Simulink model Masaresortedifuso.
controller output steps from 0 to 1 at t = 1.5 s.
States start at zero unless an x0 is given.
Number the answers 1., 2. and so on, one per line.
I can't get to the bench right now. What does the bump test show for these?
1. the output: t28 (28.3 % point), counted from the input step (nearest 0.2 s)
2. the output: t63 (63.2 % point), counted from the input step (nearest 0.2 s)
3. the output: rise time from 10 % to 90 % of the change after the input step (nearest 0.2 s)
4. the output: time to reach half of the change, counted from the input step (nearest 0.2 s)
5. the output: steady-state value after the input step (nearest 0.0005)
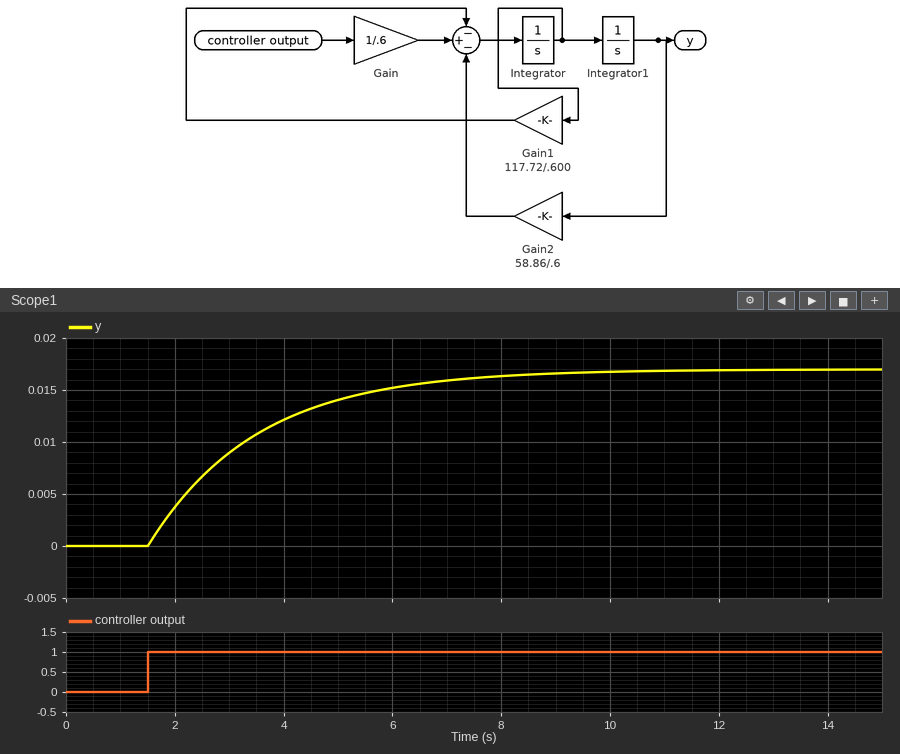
1. 0.6 s
2. 2.0 s
3. 4.4 s
4. 1.4 s
5. 0.0170
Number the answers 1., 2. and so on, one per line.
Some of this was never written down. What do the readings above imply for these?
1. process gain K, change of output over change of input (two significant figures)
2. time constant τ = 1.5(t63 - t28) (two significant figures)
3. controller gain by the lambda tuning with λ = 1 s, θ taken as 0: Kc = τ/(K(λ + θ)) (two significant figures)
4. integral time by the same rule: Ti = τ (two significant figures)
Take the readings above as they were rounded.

1. 0.017
2. 2.1 s
3. 120
4. 2.1 s
